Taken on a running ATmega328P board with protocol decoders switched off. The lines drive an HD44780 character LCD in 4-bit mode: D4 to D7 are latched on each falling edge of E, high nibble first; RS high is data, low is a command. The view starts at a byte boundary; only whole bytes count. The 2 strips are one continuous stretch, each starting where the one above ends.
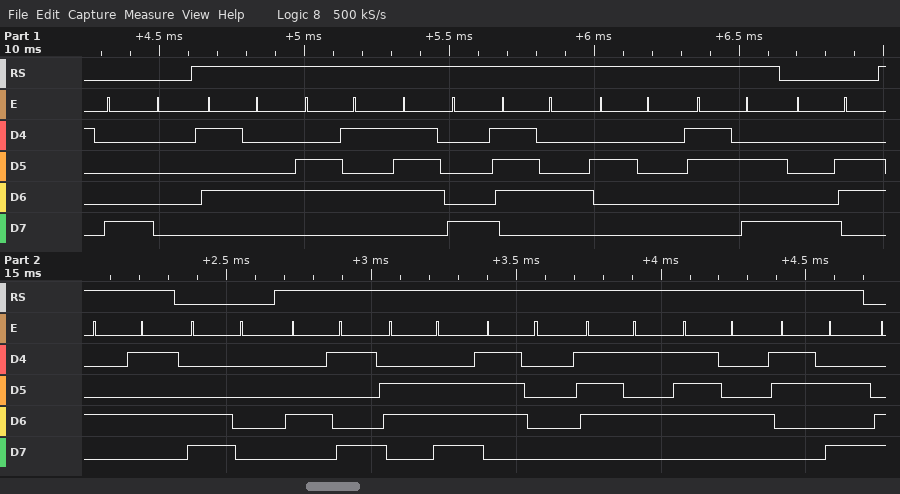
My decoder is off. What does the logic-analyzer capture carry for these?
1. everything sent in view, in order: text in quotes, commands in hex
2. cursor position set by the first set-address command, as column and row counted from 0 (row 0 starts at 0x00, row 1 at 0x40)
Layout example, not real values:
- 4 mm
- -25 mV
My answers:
- 0x80 "Text :" 0x86 "E" 0xC0 "Input:"
- column 0, row 0
